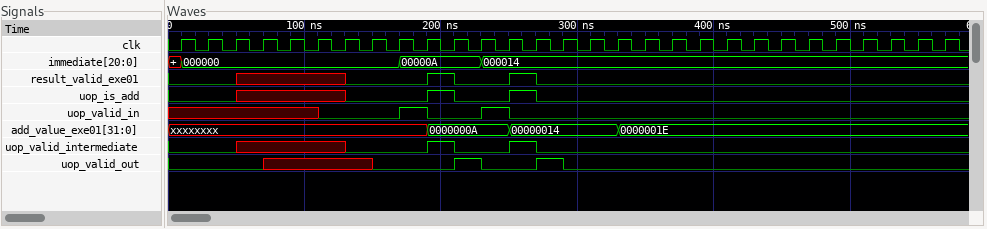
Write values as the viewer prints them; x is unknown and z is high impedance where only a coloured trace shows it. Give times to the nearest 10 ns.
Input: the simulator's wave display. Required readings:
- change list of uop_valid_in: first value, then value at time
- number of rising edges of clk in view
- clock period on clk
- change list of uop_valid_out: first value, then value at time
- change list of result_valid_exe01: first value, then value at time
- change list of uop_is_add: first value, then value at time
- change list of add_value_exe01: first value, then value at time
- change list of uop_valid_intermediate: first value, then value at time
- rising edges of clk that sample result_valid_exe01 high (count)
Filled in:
x, 0 at 110 ns, 1 at 170 ns, 0 at 190 ns, 1 at 230 ns, 0 at 250 ns
29
20 ns
0, x at 70 ns, 0 at 150 ns, 1 at 210 ns, 0 at 230 ns, 1 at 270 ns, 0 at 290 ns
0, x at 50 ns, 0 at 130 ns, 1 at 190 ns, 0 at 210 ns, 1 at 250 ns, 0 at 270 ns
0, x at 50 ns, 0 at 130 ns, 1 at 190 ns, 0 at 210 ns, 1 at 250 ns, 0 at 270 ns
xxxxxxxx, 0000000A at 190 ns, 00000014 at 250 ns, 0000001E at 330 ns
0, x at 50 ns, 0 at 130 ns, 1 at 190 ns, 0 at 210 ns, 1 at 250 ns, 0 at 270 ns
2
